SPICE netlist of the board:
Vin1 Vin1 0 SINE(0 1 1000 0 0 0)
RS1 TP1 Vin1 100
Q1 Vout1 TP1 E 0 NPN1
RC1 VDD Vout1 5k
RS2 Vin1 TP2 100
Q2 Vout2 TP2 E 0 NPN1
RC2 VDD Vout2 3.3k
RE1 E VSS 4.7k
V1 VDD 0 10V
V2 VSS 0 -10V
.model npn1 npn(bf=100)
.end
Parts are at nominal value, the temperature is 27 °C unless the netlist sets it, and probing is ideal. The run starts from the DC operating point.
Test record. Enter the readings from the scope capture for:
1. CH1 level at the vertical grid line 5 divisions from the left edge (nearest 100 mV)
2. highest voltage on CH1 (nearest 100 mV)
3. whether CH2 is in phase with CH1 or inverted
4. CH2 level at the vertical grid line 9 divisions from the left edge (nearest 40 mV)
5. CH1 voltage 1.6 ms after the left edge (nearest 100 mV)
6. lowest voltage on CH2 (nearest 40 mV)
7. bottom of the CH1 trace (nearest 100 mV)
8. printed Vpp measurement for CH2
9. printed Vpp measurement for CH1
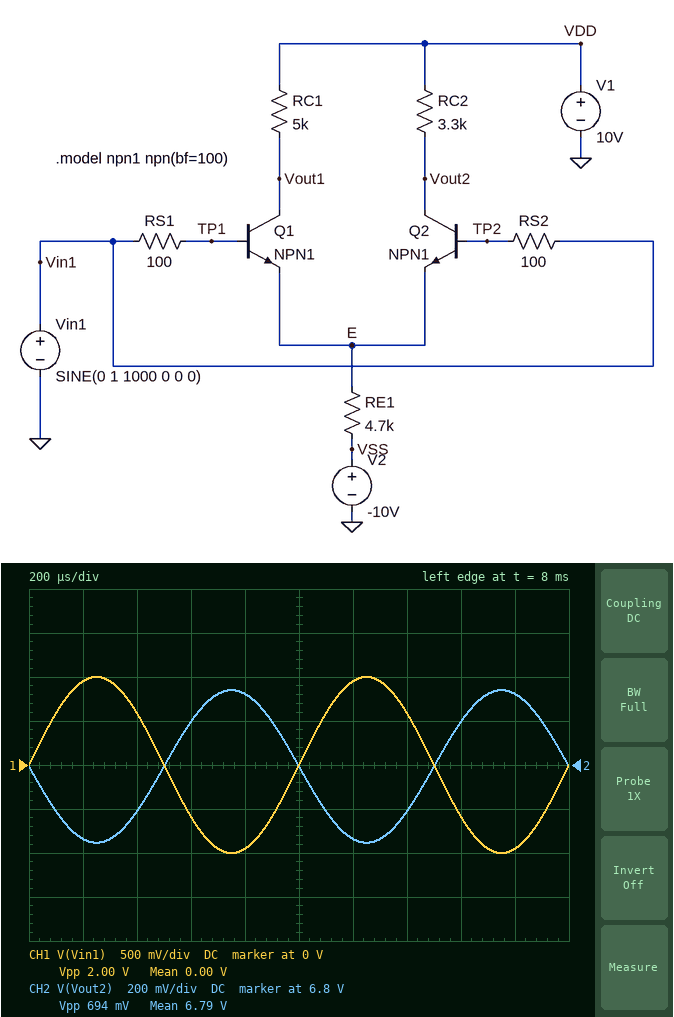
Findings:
0 V
1.0 V
inverted
7.12 V
-600 mV
6.44 V
-1.0 V
694 mV
2.00 V
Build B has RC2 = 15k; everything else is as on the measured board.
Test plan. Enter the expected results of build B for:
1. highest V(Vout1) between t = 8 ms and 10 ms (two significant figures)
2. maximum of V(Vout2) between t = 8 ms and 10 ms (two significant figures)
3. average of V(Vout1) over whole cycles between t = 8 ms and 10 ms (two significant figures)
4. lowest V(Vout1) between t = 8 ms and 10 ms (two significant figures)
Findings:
5.4 V
270 mV
4.2 V
3.1 V
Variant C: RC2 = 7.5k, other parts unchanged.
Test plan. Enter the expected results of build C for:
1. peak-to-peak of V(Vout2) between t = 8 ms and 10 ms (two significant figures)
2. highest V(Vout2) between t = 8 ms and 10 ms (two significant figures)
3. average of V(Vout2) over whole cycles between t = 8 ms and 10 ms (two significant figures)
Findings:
1.6 V
3.5 V
2.7 V
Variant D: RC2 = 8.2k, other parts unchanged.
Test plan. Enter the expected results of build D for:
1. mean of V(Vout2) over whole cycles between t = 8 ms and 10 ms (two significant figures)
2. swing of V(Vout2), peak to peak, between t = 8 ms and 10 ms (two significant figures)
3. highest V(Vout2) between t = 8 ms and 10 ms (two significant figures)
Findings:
2.0 V
1.7 V
2.9 V
